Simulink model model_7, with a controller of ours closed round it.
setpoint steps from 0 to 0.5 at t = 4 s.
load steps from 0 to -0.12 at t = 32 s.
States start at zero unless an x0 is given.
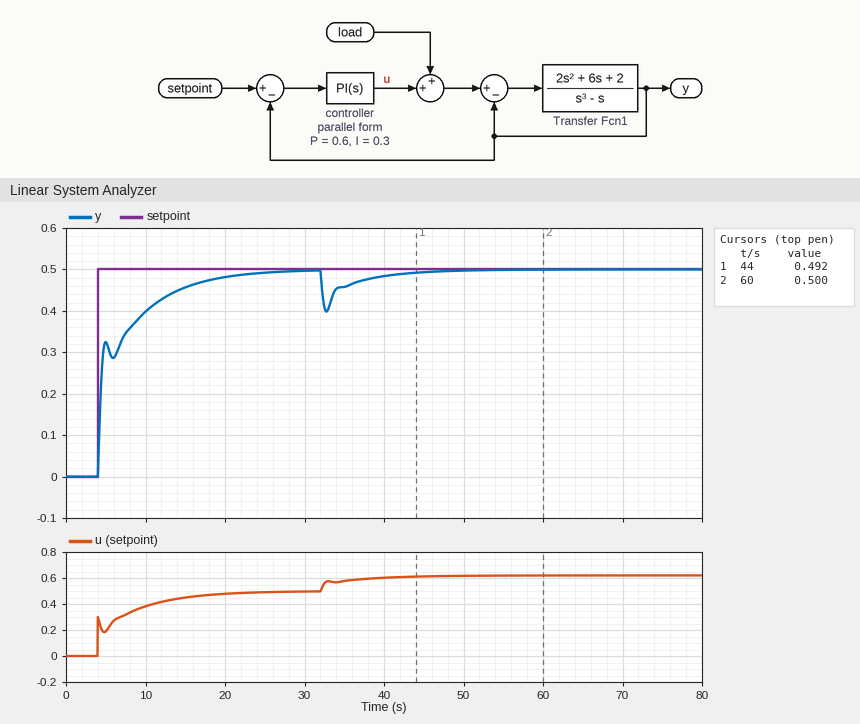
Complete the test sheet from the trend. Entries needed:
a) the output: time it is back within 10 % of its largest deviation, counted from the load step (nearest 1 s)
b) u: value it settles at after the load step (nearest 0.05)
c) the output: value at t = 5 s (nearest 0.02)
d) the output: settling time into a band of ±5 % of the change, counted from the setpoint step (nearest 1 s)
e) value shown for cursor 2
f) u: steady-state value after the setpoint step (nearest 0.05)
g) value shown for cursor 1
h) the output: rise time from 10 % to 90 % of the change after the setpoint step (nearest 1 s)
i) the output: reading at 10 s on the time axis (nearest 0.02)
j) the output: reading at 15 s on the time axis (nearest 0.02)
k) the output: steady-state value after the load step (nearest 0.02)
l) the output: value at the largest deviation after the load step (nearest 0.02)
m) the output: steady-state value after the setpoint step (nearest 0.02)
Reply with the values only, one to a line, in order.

11 s
0.60
0.32
14 s
0.500
0.50
0.492
10 s
0.40
0.46
0.50
0.40
0.50
